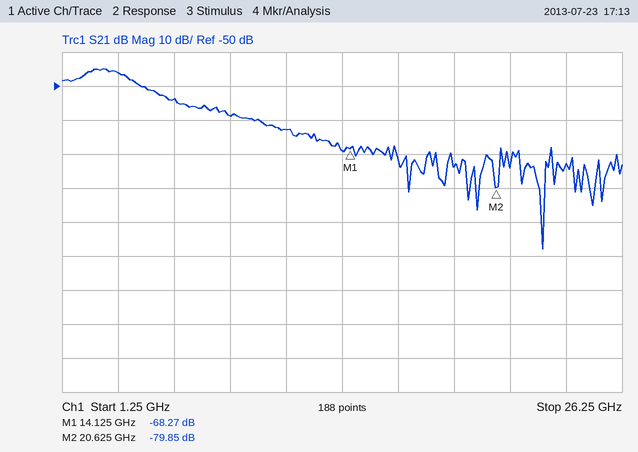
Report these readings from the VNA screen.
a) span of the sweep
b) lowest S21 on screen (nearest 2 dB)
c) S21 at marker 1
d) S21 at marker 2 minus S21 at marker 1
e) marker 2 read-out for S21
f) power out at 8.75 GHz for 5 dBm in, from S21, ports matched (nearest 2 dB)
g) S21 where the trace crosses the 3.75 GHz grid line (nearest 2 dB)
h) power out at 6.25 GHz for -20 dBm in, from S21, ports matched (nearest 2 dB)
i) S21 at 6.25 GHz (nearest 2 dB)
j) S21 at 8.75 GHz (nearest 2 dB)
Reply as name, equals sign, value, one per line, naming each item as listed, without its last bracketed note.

span of the sweep = 25 GHz
lowest S21 on screen = -98 dB
S21 at marker 1 = -68.27 dB
S21 at marker 2 minus S21 at marker 1 = -11.58 dB
marker 2 read-out for S21 = -79.85 dB
power out at 8.75 GHz for 5 dBm in, from S21, ports matched = -54 dBm
S21 where the trace crosses the 3.75 GHz grid line = -46 dB
power out at 6.25 GHz for -20 dBm in, from S21, ports matched = -74 dBm
S21 at 6.25 GHz = -54 dB
S21 at 8.75 GHz = -58 dB
